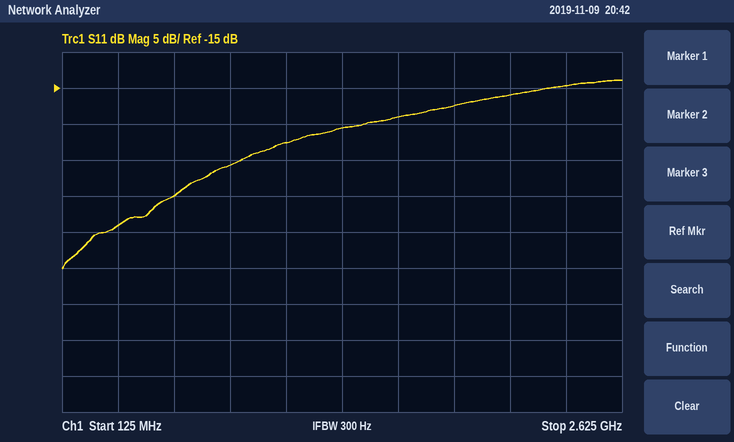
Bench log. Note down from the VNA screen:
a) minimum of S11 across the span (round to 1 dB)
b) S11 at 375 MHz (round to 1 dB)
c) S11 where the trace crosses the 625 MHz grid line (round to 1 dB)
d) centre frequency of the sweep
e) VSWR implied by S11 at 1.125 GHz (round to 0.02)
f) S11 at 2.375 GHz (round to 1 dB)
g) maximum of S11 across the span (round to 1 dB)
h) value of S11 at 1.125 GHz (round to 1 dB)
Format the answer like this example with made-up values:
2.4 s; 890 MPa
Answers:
-40 dB; -34 dB; -30 dB; 1.375 GHz; 1.16; -15 dB; -14 dB; -23 dB
